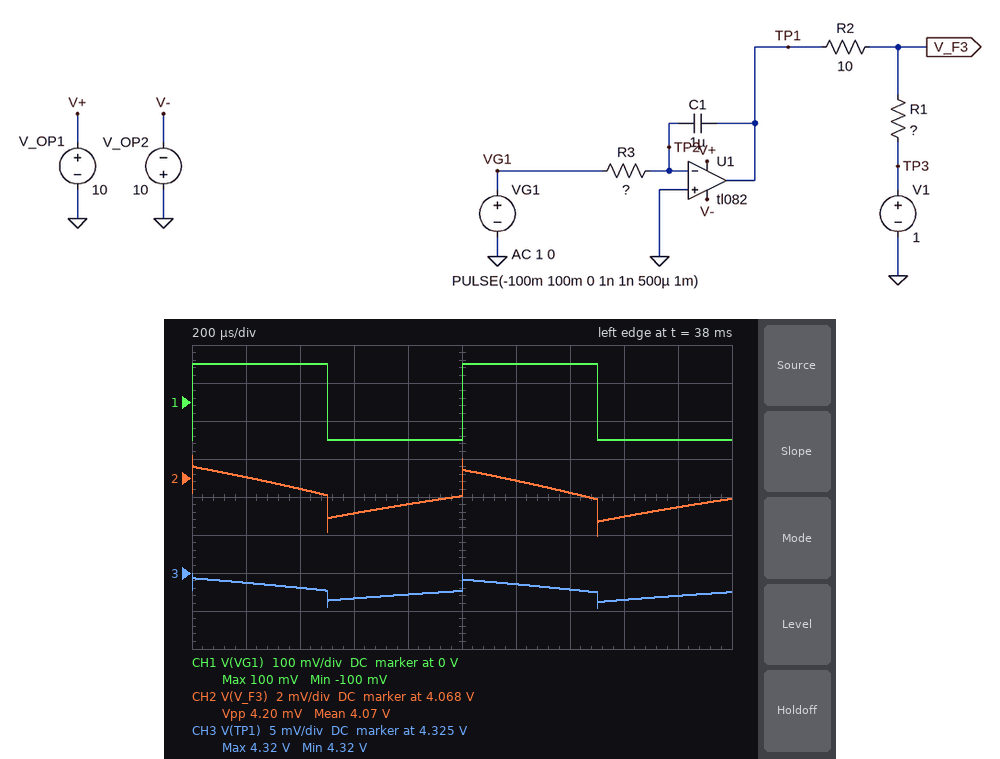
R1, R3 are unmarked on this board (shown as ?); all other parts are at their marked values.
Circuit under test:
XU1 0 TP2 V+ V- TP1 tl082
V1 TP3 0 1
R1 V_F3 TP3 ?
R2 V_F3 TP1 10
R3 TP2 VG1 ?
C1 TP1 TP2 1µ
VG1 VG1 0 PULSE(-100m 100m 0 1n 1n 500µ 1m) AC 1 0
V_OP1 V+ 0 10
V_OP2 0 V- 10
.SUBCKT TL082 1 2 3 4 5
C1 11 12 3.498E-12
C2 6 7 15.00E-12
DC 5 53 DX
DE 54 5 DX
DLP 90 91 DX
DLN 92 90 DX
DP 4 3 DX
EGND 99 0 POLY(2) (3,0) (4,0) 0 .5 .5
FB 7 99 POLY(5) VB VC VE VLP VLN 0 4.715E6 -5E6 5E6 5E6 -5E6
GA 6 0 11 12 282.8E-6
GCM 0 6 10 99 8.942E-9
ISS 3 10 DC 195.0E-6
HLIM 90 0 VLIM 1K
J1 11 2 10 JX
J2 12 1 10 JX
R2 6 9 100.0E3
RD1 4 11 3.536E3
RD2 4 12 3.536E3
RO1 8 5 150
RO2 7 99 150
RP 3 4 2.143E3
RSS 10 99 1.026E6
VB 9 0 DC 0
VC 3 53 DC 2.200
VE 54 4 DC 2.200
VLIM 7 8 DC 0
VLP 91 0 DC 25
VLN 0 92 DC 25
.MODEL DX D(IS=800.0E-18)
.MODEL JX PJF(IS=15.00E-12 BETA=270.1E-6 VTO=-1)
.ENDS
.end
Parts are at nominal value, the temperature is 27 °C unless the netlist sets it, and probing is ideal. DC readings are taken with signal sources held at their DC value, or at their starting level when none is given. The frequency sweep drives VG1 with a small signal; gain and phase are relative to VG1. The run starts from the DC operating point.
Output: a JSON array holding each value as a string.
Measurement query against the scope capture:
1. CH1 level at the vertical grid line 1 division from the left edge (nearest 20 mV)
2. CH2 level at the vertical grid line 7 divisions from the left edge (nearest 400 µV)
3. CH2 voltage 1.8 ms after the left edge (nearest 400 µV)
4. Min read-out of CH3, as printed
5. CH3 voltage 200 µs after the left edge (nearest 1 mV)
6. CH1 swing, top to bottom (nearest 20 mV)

["100 mV", "4.0672 V", "4.0664 V", "4.32 V", "4.324 V", "200 mV"]
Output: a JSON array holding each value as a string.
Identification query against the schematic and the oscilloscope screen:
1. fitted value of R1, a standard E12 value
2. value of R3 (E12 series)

["120 Ω", "12 kΩ"]
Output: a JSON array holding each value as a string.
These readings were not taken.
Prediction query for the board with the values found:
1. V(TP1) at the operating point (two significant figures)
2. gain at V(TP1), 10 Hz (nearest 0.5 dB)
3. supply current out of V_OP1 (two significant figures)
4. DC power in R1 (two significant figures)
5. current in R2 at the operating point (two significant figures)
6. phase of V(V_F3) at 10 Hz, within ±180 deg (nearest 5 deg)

["4.3 V", "-31.5 dB", "9.5 mA", "79 mW", "26 mA", "130 deg"]
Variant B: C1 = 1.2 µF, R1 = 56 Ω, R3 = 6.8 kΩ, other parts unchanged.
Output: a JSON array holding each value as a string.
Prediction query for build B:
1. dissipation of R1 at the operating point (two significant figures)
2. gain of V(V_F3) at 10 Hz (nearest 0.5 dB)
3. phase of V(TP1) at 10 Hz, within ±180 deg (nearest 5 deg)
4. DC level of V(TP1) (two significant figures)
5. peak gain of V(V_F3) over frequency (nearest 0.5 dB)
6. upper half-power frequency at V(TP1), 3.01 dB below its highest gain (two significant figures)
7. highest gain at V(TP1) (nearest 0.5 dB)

["37 mW", "-37.5 dB", "135 deg", "2.7 V", "-37.0 dB", "31 Hz", "-35.5 dB"]
